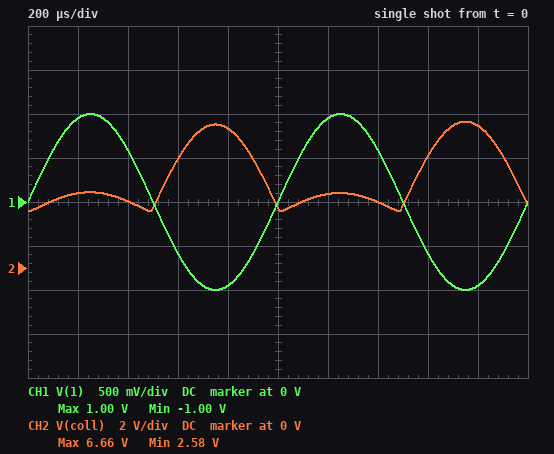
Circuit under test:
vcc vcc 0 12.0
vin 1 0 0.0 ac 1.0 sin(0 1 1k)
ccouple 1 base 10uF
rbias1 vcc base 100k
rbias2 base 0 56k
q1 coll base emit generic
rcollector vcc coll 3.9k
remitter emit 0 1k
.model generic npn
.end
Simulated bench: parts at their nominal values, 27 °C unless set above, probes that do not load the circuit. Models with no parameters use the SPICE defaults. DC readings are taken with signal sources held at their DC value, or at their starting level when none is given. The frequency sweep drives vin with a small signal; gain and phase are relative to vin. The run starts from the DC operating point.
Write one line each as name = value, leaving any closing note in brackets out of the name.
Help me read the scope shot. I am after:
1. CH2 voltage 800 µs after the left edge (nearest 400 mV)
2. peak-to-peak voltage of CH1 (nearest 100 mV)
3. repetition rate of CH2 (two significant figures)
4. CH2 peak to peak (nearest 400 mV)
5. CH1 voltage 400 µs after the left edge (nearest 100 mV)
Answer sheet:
CH2 voltage 800 µs after the left edge = 6.4 V
peak-to-peak voltage of CH1 = 2.0 V
repetition rate of CH2 = 1.0 kHz
CH2 peak to peak = 4.0 V
CH1 voltage 400 µs after the left edge = 600 mV
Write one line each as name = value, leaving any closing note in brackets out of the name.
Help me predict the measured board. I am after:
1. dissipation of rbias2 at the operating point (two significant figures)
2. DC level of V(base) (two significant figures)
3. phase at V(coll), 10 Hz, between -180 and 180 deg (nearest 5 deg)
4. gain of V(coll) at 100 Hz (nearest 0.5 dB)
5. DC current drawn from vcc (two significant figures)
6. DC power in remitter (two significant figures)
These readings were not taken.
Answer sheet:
dissipation of rbias2 at the operating point = 190 µW
DC level of V(base) = 3.2 V
phase at V(coll), 10 Hz, between -180 and 180 deg = -135 deg
gain of V(coll) at 100 Hz = 4.0 dB
DC current drawn from vcc = 2.5 mA
DC power in remitter = 6.0 mW
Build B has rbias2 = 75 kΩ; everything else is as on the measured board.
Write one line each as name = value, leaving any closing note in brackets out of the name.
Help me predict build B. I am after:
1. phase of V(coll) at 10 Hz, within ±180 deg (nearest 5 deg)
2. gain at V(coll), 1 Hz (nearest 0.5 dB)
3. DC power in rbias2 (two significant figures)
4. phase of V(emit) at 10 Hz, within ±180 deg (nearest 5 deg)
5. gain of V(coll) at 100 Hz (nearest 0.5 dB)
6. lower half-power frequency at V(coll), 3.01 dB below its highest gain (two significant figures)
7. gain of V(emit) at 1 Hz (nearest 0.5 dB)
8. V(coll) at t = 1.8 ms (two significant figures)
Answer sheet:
phase of V(coll) at 10 Hz, within ±180 deg = -125 deg
gain at V(coll), 1 Hz = -37.5 dB
DC power in rbias2 = 140 µW
phase of V(emit) at 10 Hz, within ±180 deg = 55 deg
gain of V(coll) at 100 Hz = -14.0 dB
lower half-power frequency at V(coll), 3.01 dB below its highest gain = 15 Hz
gain of V(emit) at 1 Hz = -24.0 dB
V(coll) at t = 1.8 ms = 6.4 V
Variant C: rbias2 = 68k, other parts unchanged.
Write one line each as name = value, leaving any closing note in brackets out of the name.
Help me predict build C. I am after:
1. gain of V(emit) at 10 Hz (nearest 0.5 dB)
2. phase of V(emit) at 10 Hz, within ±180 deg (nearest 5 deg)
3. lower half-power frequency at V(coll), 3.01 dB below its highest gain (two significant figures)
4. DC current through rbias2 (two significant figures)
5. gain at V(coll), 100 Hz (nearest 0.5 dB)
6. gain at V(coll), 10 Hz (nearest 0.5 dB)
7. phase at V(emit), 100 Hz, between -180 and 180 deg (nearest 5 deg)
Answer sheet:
gain of V(emit) at 10 Hz = -5.0 dB
phase of V(emit) at 10 Hz, within ±180 deg = 55 deg
lower half-power frequency at V(coll), 3.01 dB below its highest gain = 14 Hz
DC current through rbias2 = 48 µA
gain at V(coll), 100 Hz = -7.0 dB
gain at V(coll), 10 Hz = -12.0 dB
phase at V(emit), 100 Hz, between -180 and 180 deg = 10 deg
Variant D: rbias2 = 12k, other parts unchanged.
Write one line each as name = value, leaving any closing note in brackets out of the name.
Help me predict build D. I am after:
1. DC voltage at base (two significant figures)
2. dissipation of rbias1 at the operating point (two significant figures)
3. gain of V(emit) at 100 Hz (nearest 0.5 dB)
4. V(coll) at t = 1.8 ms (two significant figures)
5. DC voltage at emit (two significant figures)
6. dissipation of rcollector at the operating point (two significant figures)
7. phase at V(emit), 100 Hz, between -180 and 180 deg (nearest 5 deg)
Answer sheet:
DC voltage at base = 1.2 V
dissipation of rbias1 at the operating point = 1.2 mW
gain of V(emit) at 100 Hz = -0.5 dB
V(coll) at t = 1.8 ms = 12 V
DC voltage at emit = 480 mV
dissipation of rcollector at the operating point = 880 µW
phase at V(emit), 100 Hz, between -180 and 180 deg = 0 deg
